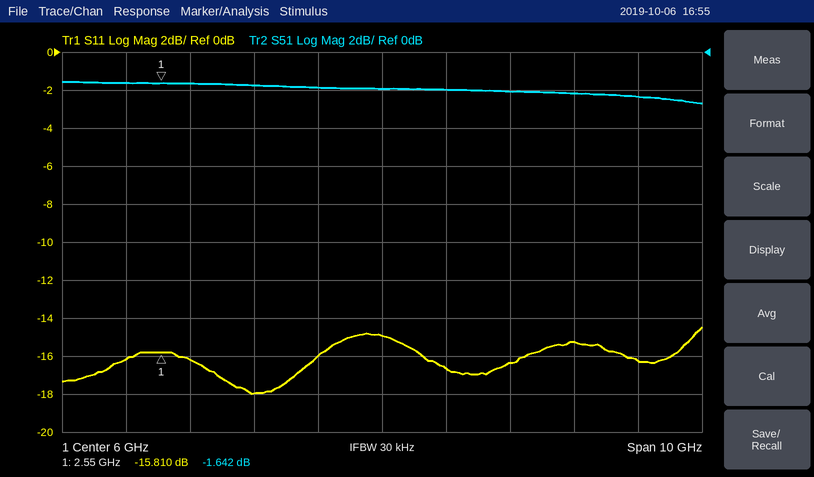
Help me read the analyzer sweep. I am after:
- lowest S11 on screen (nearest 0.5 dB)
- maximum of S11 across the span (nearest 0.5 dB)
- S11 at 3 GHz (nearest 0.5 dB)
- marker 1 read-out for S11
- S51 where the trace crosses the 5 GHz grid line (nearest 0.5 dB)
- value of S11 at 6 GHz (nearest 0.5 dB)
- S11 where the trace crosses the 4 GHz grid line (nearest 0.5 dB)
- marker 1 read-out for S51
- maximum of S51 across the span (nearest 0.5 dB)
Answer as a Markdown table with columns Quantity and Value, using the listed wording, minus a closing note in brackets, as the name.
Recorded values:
| Quantity | Value |
|---|---|
| lowest S11 on screen | -18.0 dB |
| maximum of S11 across the span | -14.5 dB |
| S11 at 3 GHz | -16.0 dB |
| marker 1 read-out for S11 | -15.810 dB |
| S51 where the trace crosses the 5 GHz grid line | -2.0 dB |
| value of S11 at 6 GHz | -15.0 dB |
| S11 where the trace crosses the 4 GHz grid line | -18.0 dB |
| marker 1 read-out for S51 | -1.642 dB |
| maximum of S51 across the span | -1.5 dB |
